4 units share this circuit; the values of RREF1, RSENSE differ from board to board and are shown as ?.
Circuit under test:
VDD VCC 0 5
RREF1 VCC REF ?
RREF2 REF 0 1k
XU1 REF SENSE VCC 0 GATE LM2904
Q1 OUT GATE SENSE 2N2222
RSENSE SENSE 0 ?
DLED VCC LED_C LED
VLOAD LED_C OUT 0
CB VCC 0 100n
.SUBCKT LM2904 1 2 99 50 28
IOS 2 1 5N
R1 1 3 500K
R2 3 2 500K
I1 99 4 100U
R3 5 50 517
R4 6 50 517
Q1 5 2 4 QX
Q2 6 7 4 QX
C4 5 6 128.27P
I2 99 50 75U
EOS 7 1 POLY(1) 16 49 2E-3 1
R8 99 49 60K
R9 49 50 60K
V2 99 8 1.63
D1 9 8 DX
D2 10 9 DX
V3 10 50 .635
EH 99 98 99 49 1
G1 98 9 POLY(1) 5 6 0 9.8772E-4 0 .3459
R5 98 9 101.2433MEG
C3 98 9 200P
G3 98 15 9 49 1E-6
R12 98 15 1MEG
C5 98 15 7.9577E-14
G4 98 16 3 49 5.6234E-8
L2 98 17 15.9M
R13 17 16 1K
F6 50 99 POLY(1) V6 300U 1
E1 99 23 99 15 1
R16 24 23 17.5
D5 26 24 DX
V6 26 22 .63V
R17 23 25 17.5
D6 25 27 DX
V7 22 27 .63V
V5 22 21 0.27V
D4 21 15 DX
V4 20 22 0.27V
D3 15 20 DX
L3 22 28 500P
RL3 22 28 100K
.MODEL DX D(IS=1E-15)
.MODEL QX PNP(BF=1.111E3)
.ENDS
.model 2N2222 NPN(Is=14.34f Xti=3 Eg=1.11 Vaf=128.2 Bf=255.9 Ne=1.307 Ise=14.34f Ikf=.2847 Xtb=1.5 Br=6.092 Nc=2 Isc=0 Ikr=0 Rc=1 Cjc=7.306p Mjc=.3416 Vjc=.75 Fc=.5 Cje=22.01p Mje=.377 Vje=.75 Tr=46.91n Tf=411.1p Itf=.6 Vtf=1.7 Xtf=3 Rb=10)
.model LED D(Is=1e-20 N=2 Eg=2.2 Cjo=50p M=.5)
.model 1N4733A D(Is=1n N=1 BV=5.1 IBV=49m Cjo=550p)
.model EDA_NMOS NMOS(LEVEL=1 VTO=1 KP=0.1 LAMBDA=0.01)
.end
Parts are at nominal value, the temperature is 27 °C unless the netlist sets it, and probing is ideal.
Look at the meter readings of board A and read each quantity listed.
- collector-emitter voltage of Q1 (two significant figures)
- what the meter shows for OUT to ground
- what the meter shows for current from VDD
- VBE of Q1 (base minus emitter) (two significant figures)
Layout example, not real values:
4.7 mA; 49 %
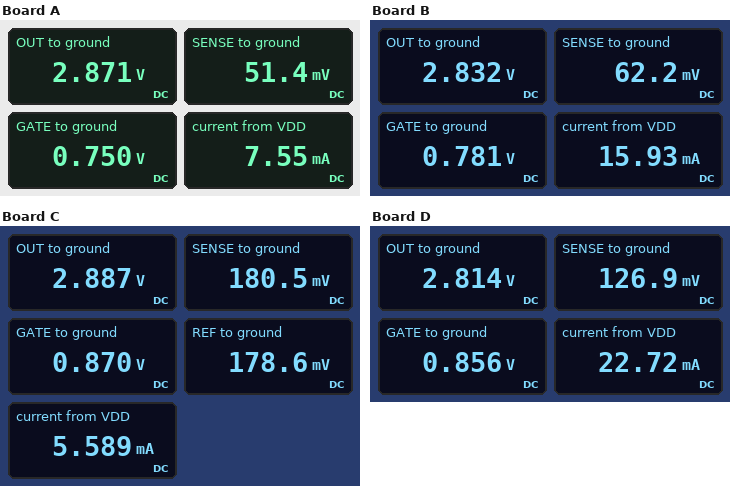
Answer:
2.8 V; 2.871 V; 7.55 mA; 700 mV
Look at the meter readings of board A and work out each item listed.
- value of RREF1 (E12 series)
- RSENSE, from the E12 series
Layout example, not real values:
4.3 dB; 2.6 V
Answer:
100 kΩ; 6.8 Ω
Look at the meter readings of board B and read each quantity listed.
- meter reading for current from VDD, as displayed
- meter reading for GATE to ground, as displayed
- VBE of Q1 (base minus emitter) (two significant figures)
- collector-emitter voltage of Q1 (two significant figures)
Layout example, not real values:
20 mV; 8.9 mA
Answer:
15.93 mA; 0.781 V; 720 mV; 2.8 V
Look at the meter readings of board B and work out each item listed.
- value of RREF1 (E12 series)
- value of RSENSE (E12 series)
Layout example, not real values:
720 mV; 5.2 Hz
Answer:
82 kΩ; 3.9 Ω
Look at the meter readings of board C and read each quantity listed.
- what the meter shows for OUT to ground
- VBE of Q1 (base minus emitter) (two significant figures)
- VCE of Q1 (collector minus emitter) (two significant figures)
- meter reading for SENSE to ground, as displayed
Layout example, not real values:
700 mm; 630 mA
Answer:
2.887 V; 690 mV; 2.7 V; 180.5 mV
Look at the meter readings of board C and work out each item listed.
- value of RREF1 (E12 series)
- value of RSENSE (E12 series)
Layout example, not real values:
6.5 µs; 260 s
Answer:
27 kΩ; 33 Ω
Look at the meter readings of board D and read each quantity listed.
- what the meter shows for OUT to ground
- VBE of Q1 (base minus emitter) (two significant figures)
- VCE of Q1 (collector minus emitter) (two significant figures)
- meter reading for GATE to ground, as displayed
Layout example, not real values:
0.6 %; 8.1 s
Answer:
2.814 V; 730 mV; 2.7 V; 0.856 V
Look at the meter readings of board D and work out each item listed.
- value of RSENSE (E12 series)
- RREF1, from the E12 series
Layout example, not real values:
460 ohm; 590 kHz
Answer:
5.6 Ω; 39 kΩ
